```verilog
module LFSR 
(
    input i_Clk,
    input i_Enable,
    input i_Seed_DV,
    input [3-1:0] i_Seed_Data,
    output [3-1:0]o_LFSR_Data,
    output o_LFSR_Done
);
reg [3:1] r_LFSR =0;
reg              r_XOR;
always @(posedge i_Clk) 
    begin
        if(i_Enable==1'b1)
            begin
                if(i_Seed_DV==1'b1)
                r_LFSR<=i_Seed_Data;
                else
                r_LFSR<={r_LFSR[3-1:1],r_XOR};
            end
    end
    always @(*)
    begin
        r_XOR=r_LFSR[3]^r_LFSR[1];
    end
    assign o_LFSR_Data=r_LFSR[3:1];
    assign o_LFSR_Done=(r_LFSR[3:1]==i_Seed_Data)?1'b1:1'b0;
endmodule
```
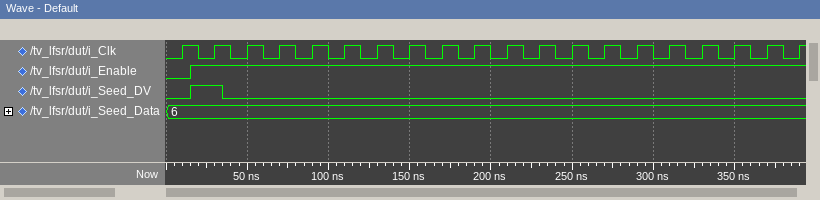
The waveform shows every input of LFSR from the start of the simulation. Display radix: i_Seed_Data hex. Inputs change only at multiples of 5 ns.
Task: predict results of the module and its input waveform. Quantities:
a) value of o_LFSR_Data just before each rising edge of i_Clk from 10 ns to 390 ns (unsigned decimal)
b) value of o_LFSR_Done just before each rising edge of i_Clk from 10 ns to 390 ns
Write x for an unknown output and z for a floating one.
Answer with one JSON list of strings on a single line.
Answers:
["0, 0, 6, 5, 2, 4, 1, 3, 7, 6, 5, 2, 4, 1, 3, 7, 6, 5, 2, 4", "0 0 1 0 0 0 0 0 0 1 0 0 0 0 0 0 1 0 0 0"]
